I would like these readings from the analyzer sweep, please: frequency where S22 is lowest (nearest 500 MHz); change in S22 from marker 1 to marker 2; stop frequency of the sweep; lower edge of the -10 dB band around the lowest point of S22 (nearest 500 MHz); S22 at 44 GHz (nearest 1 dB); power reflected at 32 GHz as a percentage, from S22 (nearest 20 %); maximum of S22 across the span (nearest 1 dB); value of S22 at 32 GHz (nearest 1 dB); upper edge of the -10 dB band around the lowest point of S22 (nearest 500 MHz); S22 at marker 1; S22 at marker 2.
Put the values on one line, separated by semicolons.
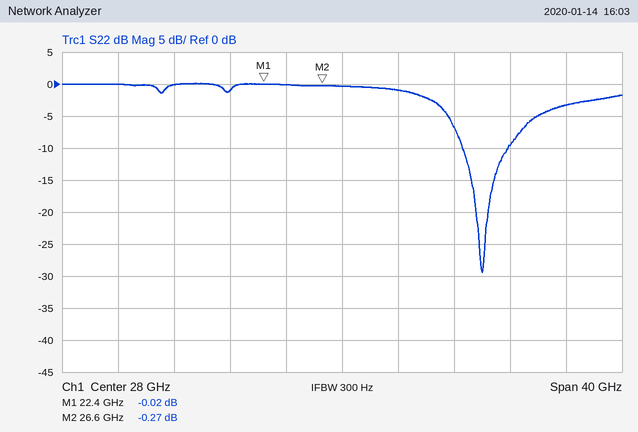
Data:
38.0 GHz; -0.25 dB; 48 GHz; 36.5 GHz; -3 dB; 80 %; 0 dB; -1 dB; 40.0 GHz; -0.02 dB; -0.27 dB
